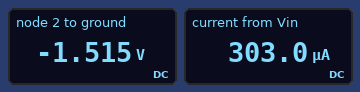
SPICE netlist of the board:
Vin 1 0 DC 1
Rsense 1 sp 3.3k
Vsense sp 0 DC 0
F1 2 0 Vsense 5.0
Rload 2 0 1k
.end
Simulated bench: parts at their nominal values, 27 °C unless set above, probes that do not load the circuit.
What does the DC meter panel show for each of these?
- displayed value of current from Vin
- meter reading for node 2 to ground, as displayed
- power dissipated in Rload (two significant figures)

303.0 µA
-1.515 V
2.3 mW
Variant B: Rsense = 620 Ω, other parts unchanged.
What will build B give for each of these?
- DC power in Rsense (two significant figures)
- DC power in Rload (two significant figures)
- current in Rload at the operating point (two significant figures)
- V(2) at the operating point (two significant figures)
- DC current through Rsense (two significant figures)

1.6 mW
65 mW
8.1 mA
-8.1 V
1.6 mA
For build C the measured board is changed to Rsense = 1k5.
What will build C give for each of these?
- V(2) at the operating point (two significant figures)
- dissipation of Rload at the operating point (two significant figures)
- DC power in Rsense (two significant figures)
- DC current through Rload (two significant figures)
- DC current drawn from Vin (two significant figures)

-3.3 V
11 mW
670 µW
3.3 mA
670 µA
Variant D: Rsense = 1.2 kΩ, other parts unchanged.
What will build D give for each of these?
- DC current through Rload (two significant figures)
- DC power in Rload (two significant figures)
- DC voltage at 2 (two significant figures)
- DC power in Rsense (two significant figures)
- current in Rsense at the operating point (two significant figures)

4.2 mA
17 mW
-4.2 V
830 µW
830 µA
